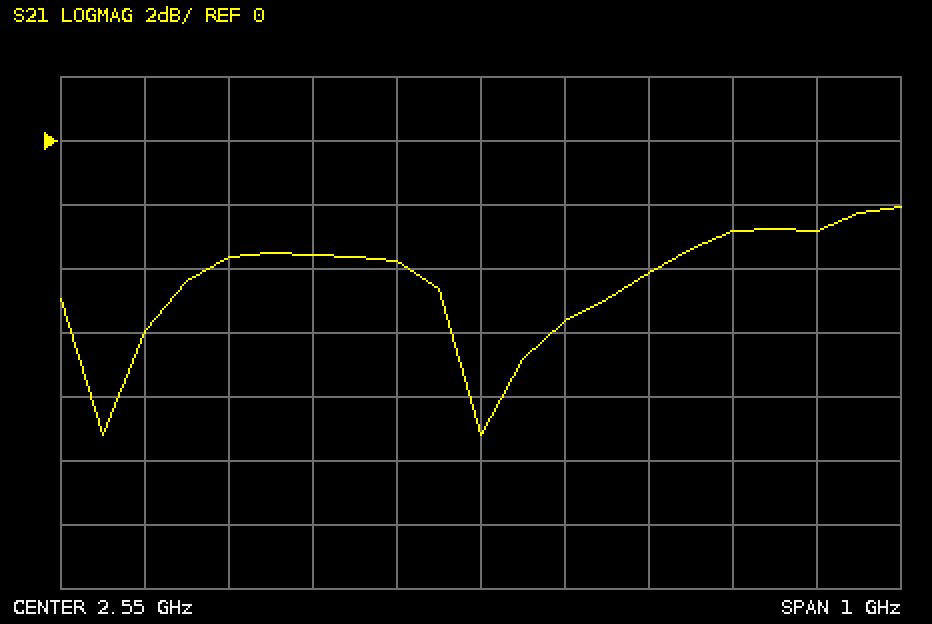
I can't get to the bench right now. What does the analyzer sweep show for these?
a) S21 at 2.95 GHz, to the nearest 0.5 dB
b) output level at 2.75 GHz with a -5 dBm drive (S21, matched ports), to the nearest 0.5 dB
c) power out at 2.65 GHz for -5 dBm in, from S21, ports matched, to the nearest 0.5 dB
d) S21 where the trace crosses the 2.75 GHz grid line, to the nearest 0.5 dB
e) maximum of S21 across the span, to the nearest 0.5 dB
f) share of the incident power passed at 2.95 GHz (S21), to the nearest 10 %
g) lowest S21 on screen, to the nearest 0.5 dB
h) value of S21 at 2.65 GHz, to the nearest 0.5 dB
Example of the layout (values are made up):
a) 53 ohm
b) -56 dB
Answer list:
a) -3.0 dB
b) -9.0 dBm
c) -10.5 dBm
d) -4.0 dB
e) -2.0 dB
f) 50 %
g) -9.0 dB
h) -5.5 dB
